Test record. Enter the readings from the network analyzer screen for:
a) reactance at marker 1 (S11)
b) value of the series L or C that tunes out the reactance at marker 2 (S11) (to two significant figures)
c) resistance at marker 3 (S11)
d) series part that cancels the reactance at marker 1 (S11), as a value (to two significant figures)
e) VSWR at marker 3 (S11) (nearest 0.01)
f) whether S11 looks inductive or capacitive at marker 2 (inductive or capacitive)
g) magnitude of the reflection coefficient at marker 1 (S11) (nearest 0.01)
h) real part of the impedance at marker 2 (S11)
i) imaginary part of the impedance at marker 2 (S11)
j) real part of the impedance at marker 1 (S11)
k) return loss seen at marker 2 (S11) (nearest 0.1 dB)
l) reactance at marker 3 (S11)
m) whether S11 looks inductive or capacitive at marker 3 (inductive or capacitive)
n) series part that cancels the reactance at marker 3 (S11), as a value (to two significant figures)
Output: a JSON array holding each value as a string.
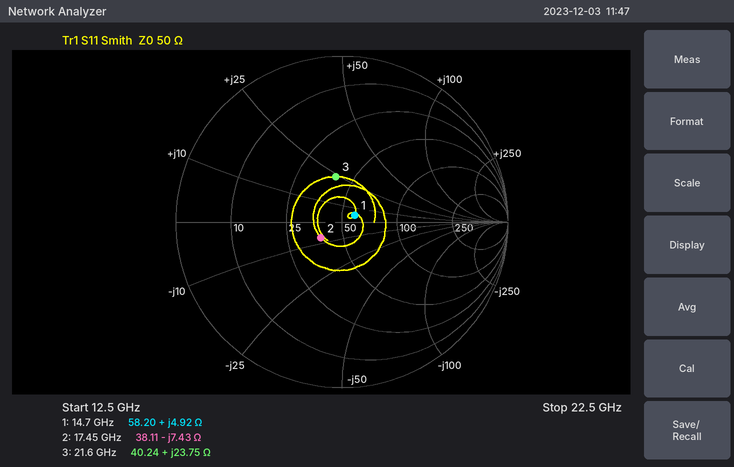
["+4.92 Ω", "68 pH", "40.24 Ω", "2.2 pF", "1.76", "capacitive", "0.09", "38.11 Ω", "-7.43 Ω", "58.20 Ω", "16.0 dB", "+23.75 Ω", "inductive", "310 fF"]
